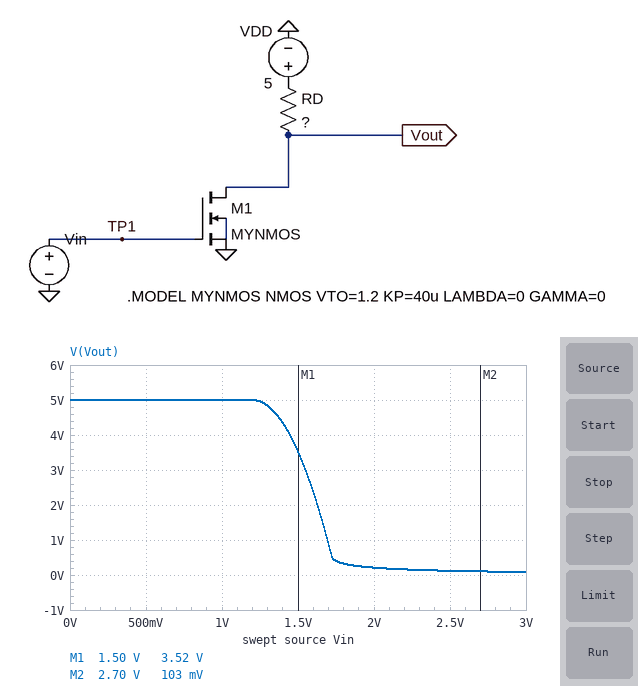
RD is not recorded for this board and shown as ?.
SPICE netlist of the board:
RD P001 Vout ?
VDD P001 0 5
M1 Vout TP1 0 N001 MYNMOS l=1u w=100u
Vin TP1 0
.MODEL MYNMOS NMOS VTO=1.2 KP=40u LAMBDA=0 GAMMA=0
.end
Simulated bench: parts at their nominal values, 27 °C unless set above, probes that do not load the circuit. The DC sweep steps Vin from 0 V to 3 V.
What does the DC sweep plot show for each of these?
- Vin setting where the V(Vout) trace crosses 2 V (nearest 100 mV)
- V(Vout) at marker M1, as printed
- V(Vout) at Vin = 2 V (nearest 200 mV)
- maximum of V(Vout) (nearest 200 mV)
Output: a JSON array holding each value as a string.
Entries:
["1.6 V", "3.52 V", "200 mV", "5.0 V"]
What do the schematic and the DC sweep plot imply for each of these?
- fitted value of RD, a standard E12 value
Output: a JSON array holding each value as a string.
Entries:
["8.2 kΩ"]
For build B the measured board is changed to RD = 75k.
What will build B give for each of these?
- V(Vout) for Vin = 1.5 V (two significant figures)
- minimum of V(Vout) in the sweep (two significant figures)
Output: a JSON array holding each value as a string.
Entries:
["61 mV", "9.3 mV"]
